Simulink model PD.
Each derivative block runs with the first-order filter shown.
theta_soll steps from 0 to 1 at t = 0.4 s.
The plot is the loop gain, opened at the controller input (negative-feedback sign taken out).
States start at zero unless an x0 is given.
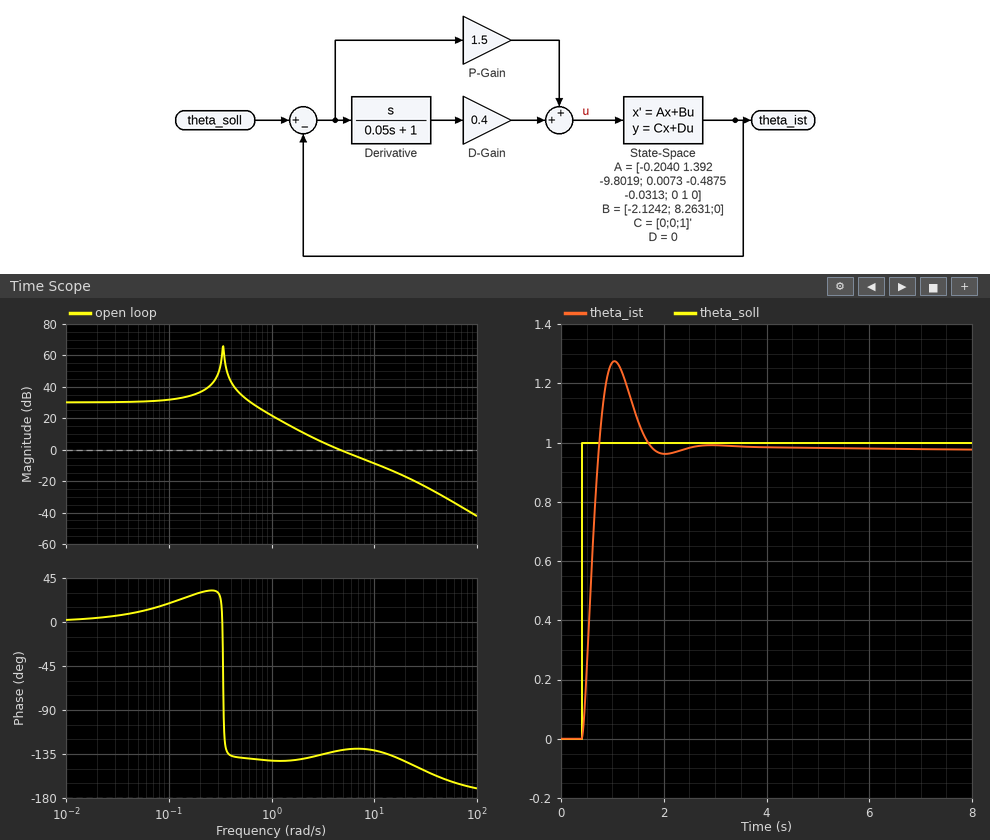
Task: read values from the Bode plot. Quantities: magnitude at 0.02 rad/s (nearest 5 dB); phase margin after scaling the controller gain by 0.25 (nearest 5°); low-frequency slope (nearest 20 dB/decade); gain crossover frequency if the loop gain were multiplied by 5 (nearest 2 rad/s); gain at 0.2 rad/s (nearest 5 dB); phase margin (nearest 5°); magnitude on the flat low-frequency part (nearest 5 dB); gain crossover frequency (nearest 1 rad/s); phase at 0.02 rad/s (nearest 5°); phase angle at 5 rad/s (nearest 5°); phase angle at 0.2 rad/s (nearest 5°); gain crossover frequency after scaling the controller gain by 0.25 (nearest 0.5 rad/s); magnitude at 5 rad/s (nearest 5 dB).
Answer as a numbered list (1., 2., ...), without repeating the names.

1. 30 dB
2. 40°
3. 0 dB/decade
4. 16 rad/s
5. 35 dB
6. 50°
7. 30 dB
8. 5 rad/s
9. 5°
10. -130°
11. 30°
12. 2.0 rad/s
13. 0 dB
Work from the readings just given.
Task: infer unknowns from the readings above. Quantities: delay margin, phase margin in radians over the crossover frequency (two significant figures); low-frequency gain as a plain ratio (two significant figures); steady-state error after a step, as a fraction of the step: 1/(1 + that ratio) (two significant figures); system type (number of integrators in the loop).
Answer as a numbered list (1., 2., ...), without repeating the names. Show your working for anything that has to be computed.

1. 50 × π / 180 / 5 = 0.17 s
2. 10^(30 / 20) = 32
3. 1 / (1 + 32) = 0.030
4. 0
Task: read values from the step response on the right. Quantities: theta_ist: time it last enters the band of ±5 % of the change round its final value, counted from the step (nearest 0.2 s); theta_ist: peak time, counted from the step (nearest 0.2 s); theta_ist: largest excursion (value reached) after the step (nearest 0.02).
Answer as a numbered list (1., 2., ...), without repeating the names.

1. 1.2 s
2. 0.6 s
3. 1.28
